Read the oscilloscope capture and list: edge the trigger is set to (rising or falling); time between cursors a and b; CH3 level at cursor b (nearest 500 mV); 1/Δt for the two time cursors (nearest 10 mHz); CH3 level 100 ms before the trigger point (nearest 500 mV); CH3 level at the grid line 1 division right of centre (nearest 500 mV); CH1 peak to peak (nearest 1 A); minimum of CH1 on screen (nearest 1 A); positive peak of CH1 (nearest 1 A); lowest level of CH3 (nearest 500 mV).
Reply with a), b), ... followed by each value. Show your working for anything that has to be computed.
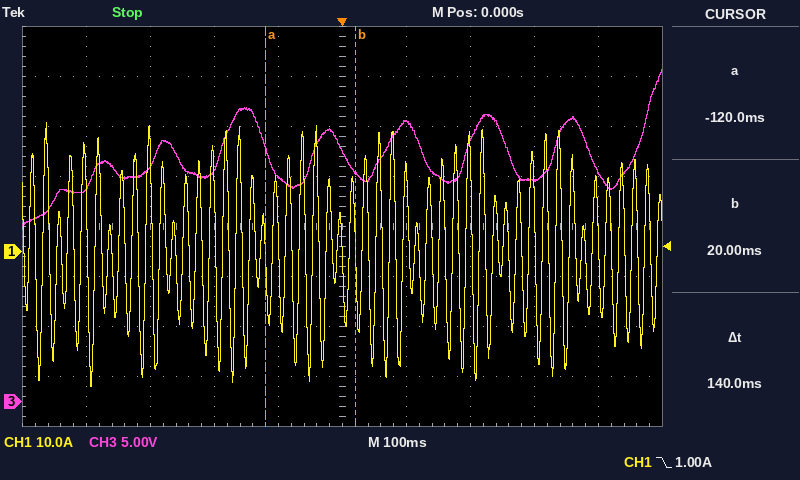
a) falling
b) 140 ms
c) 23.0 V
d) 1 / 140 ms ≈ 7.14 Hz
e) 22.5 V
f) 28.0 V
g) 26 A − (-27 A) = 53 A
h) -27 A
i) 26 A
j) 17.5 V
